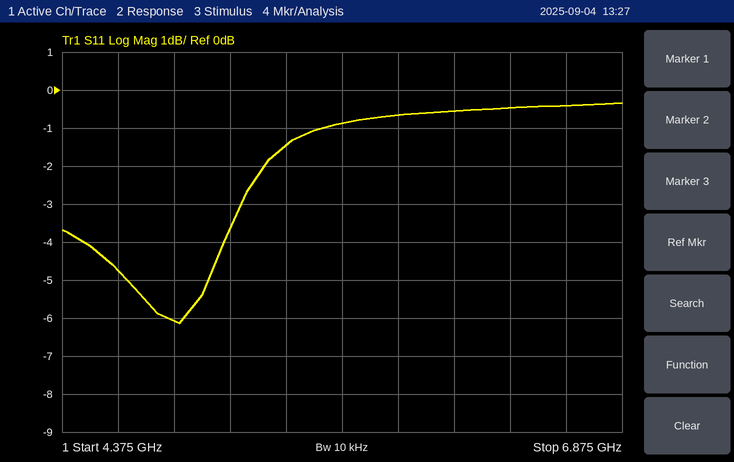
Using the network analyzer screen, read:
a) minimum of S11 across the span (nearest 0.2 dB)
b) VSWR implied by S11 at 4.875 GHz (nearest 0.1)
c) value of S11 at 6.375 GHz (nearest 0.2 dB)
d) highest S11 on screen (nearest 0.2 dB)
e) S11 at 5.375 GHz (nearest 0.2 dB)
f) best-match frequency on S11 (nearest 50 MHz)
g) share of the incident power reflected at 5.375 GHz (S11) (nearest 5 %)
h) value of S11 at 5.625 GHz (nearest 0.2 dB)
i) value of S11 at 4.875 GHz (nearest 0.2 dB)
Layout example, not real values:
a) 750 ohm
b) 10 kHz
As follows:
a) -6.2 dB
b) 3.0
c) -0.4 dB
d) -0.4 dB
e) -1.4 dB
f) 4.90 GHz
g) 70 %
h) -0.8 dB
i) -6.0 dB
